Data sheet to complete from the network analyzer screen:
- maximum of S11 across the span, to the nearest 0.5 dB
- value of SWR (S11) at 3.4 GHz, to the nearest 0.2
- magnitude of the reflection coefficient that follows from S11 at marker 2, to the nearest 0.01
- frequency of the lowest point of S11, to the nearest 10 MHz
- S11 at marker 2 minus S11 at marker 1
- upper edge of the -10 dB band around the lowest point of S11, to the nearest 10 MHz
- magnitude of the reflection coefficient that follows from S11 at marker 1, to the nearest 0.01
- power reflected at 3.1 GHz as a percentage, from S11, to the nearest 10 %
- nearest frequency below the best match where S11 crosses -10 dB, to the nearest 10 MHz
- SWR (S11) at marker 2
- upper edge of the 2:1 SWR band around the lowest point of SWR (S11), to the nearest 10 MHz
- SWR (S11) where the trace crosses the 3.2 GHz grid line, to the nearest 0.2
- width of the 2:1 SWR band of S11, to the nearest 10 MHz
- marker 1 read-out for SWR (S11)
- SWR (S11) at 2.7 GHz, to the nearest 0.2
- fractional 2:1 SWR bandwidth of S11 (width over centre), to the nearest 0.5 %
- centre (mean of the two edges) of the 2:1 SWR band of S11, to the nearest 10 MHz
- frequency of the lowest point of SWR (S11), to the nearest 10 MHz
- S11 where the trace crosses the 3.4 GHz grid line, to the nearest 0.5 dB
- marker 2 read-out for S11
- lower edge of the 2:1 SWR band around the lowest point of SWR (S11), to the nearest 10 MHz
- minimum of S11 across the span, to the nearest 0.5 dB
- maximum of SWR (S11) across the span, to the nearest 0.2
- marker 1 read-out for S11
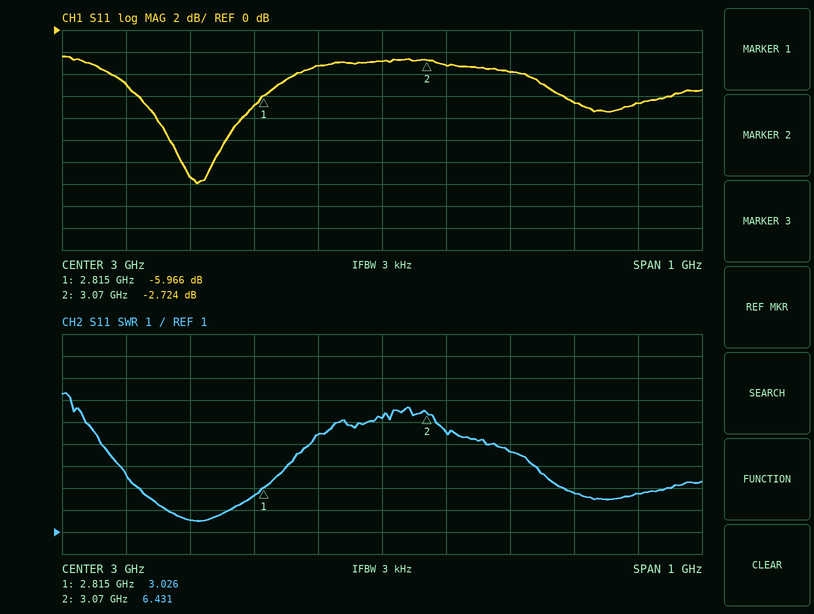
-2.5 dB
2.8
0.73
2.71 GHz
3.242 dB
2.76 GHz
0.50
50 %
2.67 GHz
6.431
2.76 GHz
4.6
100 MHz
3.026
1.6
3.5 %
2.71 GHz
2.71 GHz
-6.5 dB
-2.724 dB
2.66 GHz
-14.0 dB
7.4
-5.966 dB
